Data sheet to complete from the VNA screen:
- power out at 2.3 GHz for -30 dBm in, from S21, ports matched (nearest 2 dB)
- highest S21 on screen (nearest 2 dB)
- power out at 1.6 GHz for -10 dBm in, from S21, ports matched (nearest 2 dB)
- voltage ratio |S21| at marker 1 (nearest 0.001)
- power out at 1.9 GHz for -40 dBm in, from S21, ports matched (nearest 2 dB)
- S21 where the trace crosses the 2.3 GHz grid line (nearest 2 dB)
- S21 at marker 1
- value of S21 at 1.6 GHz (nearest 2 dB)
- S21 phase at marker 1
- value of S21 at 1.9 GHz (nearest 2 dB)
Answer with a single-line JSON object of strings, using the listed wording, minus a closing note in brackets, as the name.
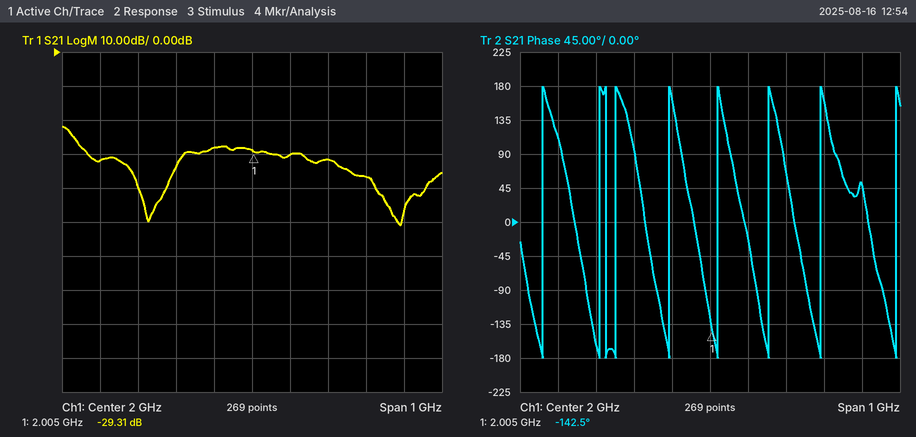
{"power out at 2.3 GHz for -30 dBm in, from S21, ports matched": "-66 dBm", "highest S21 on screen": "-22 dB", "power out at 1.6 GHz for -10 dBm in, from S21, ports matched": "-42 dBm", "voltage ratio |S21| at marker 1": "0.034", "power out at 1.9 GHz for -40 dBm in, from S21, ports matched": "-68 dBm", "S21 where the trace crosses the 2.3 GHz grid line": "-36 dB", "S21 at marker 1": "-29.31 dB", "value of S21 at 1.6 GHz": "-32 dB", "S21 phase at marker 1": "-142.5°", "value of S21 at 1.9 GHz": "-28 dB"}
